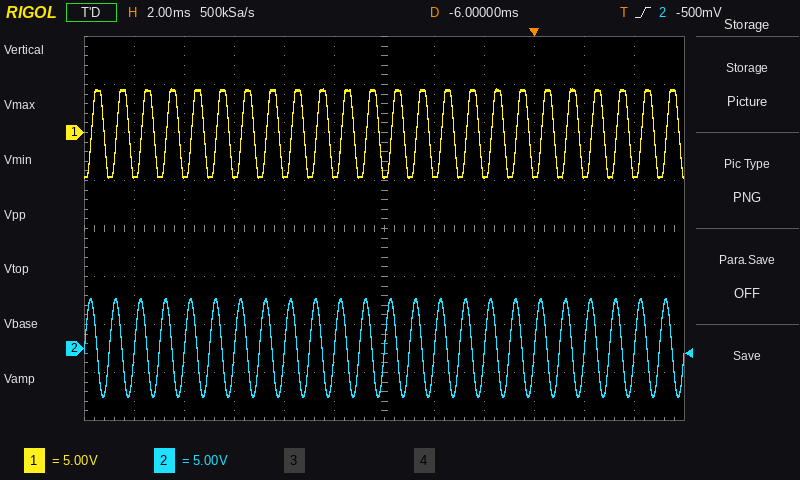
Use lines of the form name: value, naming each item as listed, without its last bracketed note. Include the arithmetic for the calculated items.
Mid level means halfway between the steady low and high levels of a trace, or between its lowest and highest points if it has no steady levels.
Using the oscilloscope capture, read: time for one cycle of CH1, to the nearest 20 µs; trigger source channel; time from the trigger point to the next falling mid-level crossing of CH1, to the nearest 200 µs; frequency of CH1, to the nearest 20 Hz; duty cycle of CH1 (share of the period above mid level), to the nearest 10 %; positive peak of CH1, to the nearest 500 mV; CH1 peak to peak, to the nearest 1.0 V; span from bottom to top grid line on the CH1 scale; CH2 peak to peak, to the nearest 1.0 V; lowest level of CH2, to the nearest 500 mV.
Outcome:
time for one cycle of CH1, to the nearest 20 µs: 1.00 ms
trigger source channel: CH2
time from the trigger point to the next falling mid-level crossing of CH1, to the nearest 200 µs: 800 µs
frequency of CH1, to the nearest 20 Hz: 1 / 1.00 ms ≈ 1.00 kHz
duty cycle of CH1 (share of the period above mid level), to the nearest 10 %: 50 %
positive peak of CH1, to the nearest 500 mV: 4.5 V
CH1 peak to peak, to the nearest 1.0 V: 9.0 V
span from bottom to top grid line on the CH1 scale: 40 V
CH2 peak to peak, to the nearest 1.0 V: 10.0 V
lowest level of CH2, to the nearest 500 mV: -5.0 V
